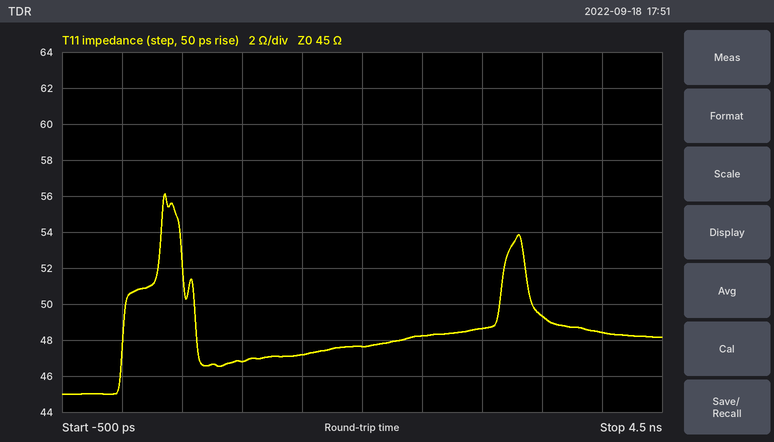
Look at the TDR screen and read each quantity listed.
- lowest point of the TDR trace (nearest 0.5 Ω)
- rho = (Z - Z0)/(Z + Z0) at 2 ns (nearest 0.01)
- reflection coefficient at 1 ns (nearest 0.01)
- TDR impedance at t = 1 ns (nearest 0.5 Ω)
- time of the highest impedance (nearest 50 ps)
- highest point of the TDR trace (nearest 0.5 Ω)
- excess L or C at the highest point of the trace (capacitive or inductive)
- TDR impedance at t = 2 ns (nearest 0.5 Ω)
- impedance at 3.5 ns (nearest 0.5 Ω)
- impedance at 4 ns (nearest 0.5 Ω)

45.0 Ω
+0.03
+0.02
47.0 Ω
350 ps
56.0 Ω
inductive
47.5 Ω
49.5 Ω
48.5 Ω
